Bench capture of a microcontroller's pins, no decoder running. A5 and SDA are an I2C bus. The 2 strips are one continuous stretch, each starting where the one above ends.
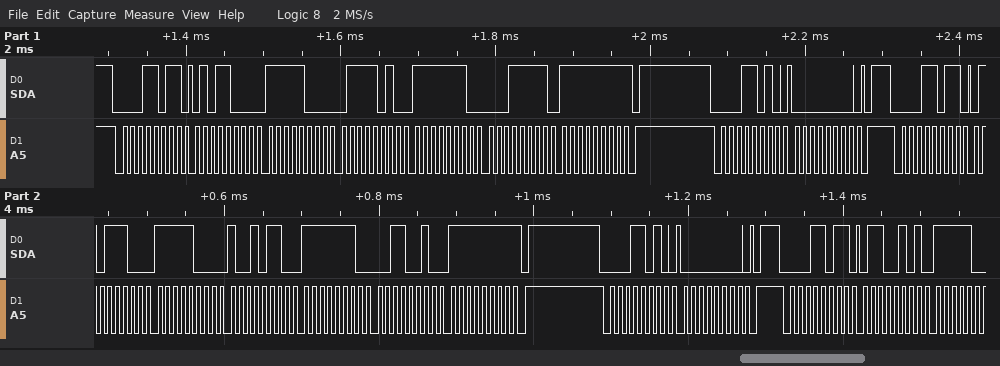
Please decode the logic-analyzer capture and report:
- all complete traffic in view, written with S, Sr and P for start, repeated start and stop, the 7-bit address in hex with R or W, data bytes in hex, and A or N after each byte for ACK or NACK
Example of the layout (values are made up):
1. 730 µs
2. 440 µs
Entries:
1. S 0DR A 58 A F8 A 7A A FE A 1F A FF N P S 0DW A 00 A P S 0DR A 5C A F8 A 96 A FE A 32 A FF N P S 0DW A 00 A P S 0DR A 65 A
